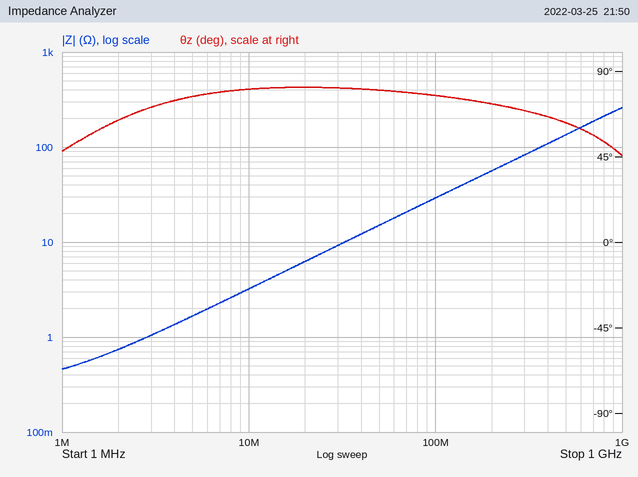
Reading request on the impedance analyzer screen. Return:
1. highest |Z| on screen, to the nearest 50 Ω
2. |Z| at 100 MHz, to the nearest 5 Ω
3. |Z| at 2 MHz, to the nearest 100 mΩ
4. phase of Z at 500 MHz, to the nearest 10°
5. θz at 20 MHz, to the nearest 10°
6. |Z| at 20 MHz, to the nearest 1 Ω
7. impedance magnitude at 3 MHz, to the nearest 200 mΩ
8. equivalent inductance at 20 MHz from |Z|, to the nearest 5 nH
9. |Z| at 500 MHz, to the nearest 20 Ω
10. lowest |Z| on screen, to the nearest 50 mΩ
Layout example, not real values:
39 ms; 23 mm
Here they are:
250 Ω; 30 Ω; 700 mΩ; 60°; 80°; 6 Ω; 1.0 Ω; 50 nH; 140 Ω; 450 mΩ
